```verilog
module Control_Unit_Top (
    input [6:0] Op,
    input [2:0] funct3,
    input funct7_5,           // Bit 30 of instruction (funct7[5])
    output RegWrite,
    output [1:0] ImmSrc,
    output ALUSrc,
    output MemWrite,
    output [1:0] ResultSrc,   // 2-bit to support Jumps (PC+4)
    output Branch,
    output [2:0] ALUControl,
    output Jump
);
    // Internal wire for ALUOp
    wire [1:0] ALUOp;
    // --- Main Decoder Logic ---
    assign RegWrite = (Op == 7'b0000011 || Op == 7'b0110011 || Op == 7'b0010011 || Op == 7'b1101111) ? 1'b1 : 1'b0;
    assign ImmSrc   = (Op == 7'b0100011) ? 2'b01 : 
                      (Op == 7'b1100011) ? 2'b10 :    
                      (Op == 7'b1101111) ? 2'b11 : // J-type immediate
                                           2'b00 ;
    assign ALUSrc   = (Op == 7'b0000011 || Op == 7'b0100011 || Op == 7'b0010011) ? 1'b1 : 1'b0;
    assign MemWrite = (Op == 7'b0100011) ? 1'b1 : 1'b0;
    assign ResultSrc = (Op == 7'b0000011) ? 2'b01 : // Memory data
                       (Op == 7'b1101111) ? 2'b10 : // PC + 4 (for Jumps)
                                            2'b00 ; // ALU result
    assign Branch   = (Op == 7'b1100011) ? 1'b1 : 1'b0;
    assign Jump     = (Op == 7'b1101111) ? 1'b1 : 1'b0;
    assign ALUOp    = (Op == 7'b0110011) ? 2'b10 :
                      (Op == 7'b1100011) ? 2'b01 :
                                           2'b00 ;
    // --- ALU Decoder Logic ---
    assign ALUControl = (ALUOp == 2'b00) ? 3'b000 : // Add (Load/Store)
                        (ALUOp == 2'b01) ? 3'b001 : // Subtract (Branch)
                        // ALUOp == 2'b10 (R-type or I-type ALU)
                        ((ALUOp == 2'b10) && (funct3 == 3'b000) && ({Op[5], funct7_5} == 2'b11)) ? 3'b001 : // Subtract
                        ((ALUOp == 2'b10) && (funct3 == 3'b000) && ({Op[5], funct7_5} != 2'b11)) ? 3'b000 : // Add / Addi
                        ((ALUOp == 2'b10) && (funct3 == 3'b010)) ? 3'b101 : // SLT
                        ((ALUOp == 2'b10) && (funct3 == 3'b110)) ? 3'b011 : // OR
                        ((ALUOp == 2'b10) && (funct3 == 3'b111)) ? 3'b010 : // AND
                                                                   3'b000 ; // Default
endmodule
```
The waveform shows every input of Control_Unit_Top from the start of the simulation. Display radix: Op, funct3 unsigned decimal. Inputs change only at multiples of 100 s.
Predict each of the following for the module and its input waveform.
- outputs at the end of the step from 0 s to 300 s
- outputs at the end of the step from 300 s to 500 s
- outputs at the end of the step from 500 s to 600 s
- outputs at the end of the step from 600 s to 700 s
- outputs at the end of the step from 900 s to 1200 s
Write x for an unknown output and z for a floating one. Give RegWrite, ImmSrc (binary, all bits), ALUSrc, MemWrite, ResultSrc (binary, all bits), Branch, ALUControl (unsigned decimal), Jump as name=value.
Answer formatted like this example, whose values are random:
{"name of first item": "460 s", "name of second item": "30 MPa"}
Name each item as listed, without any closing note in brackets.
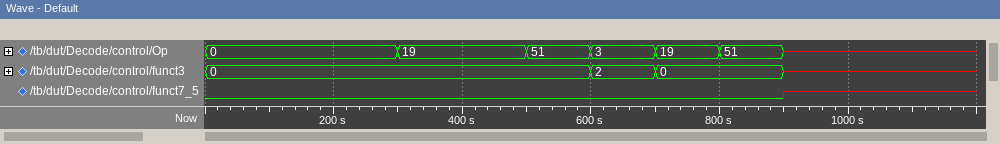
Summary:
{"outputs at the end of the step from 0 s to 300 s": "RegWrite=0, ImmSrc=00, ALUSrc=0, MemWrite=0, ResultSrc=00, Branch=0, ALUControl=0, Jump=0", "outputs at the end of the step from 300 s to 500 s": "RegWrite=1, ImmSrc=00, ALUSrc=1, MemWrite=0, ResultSrc=00, Branch=0, ALUControl=0, Jump=0", "outputs at the end of the step from 500 s to 600 s": "RegWrite=1, ImmSrc=00, ALUSrc=0, MemWrite=0, ResultSrc=00, Branch=0, ALUControl=0, Jump=0", "outputs at the end of the step from 600 s to 700 s": "RegWrite=1, ImmSrc=00, ALUSrc=1, MemWrite=0, ResultSrc=01, Branch=0, ALUControl=0, Jump=0", "outputs at the end of the step from 900 s to 1200 s": "RegWrite=x, ImmSrc=x, ALUSrc=x, MemWrite=x, ResultSrc=x, Branch=x, ALUControl=x, Jump=x"}
